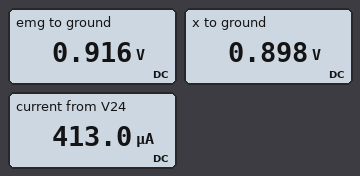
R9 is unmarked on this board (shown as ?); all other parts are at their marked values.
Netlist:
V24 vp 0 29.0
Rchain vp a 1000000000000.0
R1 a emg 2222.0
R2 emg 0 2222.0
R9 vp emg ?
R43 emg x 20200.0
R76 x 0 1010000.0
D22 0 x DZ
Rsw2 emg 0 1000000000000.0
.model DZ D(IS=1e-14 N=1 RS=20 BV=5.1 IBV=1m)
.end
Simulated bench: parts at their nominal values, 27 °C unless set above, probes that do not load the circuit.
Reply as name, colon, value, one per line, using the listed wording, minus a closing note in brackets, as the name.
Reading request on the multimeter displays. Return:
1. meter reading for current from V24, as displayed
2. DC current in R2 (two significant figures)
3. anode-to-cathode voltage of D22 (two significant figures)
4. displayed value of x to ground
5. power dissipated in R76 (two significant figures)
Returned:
meter reading for current from V24, as displayed: 413.0 µA
DC current in R2: 410 µA
anode-to-cathode voltage of D22: -900 mV
displayed value of x to ground: 0.898 V
power dissipated in R76: 800 nW
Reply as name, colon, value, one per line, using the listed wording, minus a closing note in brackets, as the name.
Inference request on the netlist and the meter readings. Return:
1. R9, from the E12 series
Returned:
R9, from the E12 series: 68 kΩ
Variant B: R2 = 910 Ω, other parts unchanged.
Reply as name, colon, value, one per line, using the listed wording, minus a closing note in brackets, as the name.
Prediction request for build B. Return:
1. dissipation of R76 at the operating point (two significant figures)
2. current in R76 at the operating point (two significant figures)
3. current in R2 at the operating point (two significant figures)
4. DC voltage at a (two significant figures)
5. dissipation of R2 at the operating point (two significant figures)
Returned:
dissipation of R76 at the operating point: 140 nW
current in R76 at the operating point: 370 nA
current in R2 at the operating point: 420 µA
DC voltage at a: 380 mV
dissipation of R2 at the operating point: 160 µW
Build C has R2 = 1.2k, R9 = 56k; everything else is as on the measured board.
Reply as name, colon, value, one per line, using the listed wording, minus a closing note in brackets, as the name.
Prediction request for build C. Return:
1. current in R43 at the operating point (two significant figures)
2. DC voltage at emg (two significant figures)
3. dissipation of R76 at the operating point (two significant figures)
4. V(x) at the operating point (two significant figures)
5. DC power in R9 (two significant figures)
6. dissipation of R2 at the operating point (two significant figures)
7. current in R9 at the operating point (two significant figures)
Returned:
current in R43 at the operating point: 590 nA
DC voltage at emg: 610 mV
dissipation of R76 at the operating point: 350 nW
V(x) at the operating point: 600 mV
DC power in R9: 14 mW
dissipation of R2 at the operating point: 310 µW
current in R9 at the operating point: 510 µA
